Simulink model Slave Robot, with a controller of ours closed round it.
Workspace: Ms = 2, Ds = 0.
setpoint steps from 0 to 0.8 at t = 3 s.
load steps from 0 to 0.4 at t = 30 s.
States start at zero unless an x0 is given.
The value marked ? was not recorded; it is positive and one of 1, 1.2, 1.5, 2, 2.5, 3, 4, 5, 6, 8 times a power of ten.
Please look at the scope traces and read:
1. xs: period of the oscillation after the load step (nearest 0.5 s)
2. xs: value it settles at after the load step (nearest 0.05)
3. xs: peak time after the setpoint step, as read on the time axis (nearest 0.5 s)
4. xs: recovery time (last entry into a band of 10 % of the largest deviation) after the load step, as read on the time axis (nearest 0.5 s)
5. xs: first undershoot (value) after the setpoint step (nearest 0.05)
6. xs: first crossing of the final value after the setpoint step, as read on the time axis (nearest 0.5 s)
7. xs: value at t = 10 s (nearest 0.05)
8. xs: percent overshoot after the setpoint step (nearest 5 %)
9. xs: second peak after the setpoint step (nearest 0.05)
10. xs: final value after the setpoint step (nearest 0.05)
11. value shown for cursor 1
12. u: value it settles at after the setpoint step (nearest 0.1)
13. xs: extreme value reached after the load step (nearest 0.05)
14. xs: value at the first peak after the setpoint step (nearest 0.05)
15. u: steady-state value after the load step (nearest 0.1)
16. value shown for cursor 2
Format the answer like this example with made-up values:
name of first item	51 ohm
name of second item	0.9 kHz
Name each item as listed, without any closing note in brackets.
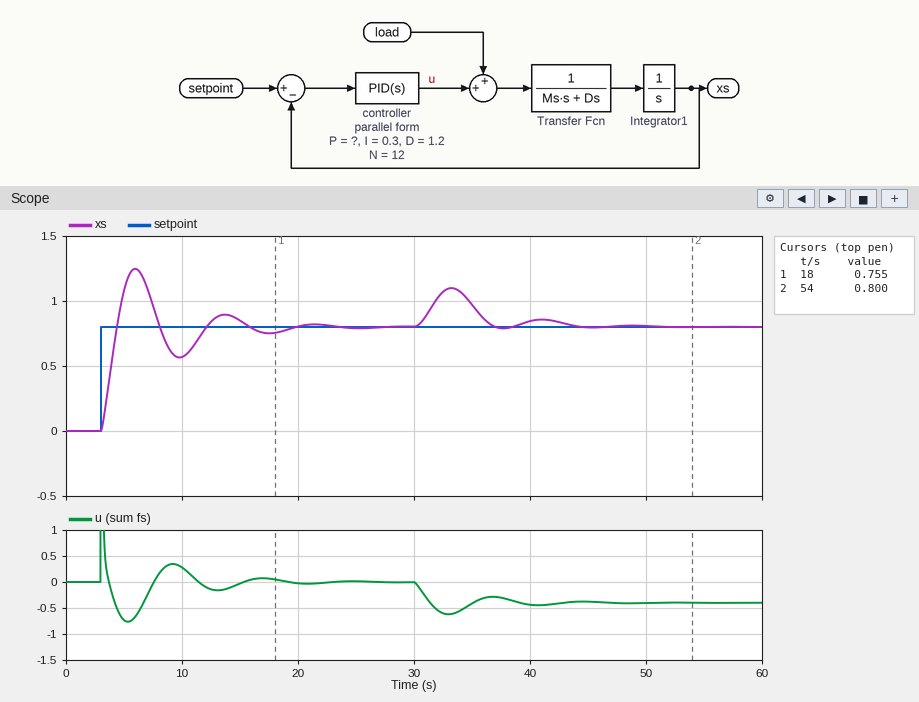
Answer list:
xs: period of the oscillation after the load step	8.0 s
xs: value it settles at after the load step	0.80
xs: peak time after the setpoint step, as read on the time axis	6.0 s
xs: recovery time (last entry into a band of 10 % of the largest deviation) after the load step, as read on the time axis	43.0 s
xs: first undershoot (value) after the setpoint step	0.55
xs: first crossing of the final value after the setpoint step, as read on the time axis	4.5 s
xs: value at t = 10 s	0.55
xs: percent overshoot after the setpoint step	55 %
xs: second peak after the setpoint step	0.90
xs: final value after the setpoint step	0.80
value shown for cursor 1	0.755
u: value it settles at after the setpoint step	0.0
xs: extreme value reached after the load step	1.10
xs: value at the first peak after the setpoint step	1.25
u: steady-state value after the load step	-0.4
value shown for cursor 2	0.800
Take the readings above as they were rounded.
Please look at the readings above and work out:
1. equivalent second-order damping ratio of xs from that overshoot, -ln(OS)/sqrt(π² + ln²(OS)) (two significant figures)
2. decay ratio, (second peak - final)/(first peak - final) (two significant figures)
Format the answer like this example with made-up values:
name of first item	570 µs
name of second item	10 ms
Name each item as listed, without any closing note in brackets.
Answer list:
equivalent second-order damping ratio of xs from that overshoot, -ln(OS)/sqrt(π² + ln²(OS))	0.19
decay ratio, (second peak - final)/(first peak - final)	0.22
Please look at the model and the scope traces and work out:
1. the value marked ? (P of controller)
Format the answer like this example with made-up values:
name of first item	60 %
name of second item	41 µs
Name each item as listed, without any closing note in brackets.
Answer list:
the value marked ?	1.5
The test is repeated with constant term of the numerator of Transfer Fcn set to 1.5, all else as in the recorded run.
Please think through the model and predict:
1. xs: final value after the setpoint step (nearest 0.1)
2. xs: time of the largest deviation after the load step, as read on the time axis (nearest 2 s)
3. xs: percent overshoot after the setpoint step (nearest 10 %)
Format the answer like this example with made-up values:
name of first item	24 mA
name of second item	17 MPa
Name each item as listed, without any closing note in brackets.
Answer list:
xs: final value after the setpoint step	0.8
xs: time of the largest deviation after the load step, as read on the time axis	32 s
xs: percent overshoot after the setpoint step	50 %
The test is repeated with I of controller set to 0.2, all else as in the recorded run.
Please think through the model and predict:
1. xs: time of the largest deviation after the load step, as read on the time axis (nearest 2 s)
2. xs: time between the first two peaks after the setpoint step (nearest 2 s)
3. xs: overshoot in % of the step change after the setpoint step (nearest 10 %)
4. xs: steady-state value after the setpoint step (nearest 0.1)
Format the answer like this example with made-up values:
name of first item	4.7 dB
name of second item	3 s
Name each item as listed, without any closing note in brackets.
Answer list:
xs: time of the largest deviation after the load step, as read on the time axis	34 s
xs: time between the first two peaks after the setpoint step	8 s
xs: overshoot in % of the step change after the setpoint step	50 %
xs: steady-state value after the setpoint step	0.8
